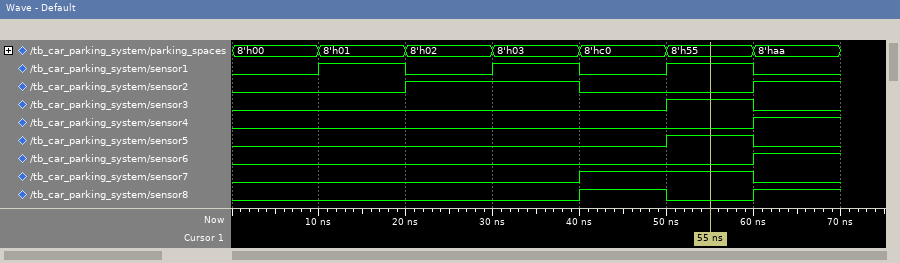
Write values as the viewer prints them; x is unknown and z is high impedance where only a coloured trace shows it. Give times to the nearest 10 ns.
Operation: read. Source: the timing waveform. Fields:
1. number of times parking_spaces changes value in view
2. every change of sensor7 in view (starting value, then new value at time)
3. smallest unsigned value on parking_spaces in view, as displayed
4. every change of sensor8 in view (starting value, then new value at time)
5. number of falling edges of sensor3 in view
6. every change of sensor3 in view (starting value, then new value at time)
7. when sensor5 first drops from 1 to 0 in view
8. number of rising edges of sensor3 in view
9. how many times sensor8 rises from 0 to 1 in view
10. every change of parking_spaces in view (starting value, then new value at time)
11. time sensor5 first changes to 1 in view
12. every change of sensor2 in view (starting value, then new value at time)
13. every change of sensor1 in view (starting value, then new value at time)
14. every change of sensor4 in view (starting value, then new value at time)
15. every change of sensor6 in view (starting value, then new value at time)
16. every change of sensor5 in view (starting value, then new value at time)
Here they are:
6
0, 1 at 40 ns, 0 at 60 ns
8'h00
0, 1 at 40 ns, 0 at 50 ns, 1 at 60 ns
1
0, 1 at 50 ns, 0 at 60 ns
60 ns
1
2
8'h00, 8'h01 at 10 ns, 8'h02 at 20 ns, 8'h03 at 30 ns, 8'hc0 at 40 ns, 8'h55 at 50 ns, 8'haa at 60 ns
50 ns
0, 1 at 20 ns, 0 at 40 ns, 1 at 60 ns
0, 1 at 10 ns, 0 at 20 ns, 1 at 30 ns, 0 at 40 ns, 1 at 50 ns, 0 at 60 ns
0, 1 at 60 ns
0, 1 at 60 ns
0, 1 at 50 ns, 0 at 60 ns
